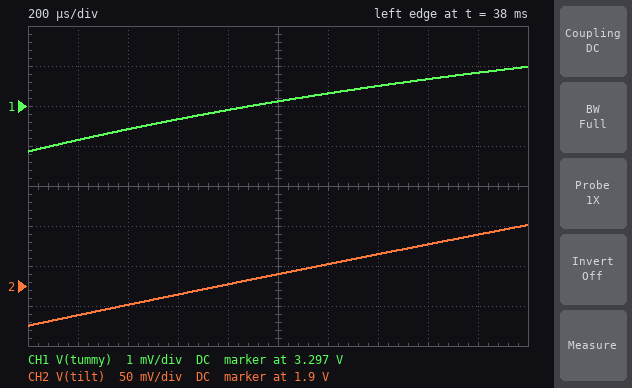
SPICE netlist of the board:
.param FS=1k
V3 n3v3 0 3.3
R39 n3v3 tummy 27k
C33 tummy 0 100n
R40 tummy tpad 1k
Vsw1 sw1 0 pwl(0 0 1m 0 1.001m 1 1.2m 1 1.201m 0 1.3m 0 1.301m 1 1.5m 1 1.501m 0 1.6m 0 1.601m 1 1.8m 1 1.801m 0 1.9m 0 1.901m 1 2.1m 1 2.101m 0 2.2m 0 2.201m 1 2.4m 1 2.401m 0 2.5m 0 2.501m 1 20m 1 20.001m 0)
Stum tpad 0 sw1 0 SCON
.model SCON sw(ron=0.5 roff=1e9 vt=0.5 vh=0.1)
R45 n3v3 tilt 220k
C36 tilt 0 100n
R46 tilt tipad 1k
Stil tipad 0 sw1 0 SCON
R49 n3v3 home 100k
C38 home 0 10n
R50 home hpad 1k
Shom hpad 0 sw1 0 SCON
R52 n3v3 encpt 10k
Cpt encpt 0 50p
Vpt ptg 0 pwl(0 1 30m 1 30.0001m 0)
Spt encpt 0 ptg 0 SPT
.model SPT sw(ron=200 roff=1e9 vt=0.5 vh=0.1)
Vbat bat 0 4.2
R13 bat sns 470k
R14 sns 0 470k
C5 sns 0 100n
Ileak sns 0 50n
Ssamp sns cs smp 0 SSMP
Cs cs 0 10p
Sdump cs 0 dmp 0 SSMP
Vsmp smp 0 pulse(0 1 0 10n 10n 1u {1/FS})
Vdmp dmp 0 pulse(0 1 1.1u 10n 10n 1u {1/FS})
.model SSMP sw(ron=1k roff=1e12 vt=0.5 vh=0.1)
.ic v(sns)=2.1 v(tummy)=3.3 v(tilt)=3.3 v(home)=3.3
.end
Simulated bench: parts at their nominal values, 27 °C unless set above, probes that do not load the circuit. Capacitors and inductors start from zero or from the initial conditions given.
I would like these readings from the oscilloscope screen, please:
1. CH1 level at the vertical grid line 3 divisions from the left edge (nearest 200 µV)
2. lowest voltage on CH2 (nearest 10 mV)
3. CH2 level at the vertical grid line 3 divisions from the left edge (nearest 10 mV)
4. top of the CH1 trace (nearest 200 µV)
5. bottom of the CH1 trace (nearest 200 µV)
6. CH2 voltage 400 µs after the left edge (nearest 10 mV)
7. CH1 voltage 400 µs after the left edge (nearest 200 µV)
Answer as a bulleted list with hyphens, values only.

- 3.2966 V
- 1.85 V
- 1.89 V
- 3.2980 V
- 3.2958 V
- 1.88 V
- 3.2964 V
